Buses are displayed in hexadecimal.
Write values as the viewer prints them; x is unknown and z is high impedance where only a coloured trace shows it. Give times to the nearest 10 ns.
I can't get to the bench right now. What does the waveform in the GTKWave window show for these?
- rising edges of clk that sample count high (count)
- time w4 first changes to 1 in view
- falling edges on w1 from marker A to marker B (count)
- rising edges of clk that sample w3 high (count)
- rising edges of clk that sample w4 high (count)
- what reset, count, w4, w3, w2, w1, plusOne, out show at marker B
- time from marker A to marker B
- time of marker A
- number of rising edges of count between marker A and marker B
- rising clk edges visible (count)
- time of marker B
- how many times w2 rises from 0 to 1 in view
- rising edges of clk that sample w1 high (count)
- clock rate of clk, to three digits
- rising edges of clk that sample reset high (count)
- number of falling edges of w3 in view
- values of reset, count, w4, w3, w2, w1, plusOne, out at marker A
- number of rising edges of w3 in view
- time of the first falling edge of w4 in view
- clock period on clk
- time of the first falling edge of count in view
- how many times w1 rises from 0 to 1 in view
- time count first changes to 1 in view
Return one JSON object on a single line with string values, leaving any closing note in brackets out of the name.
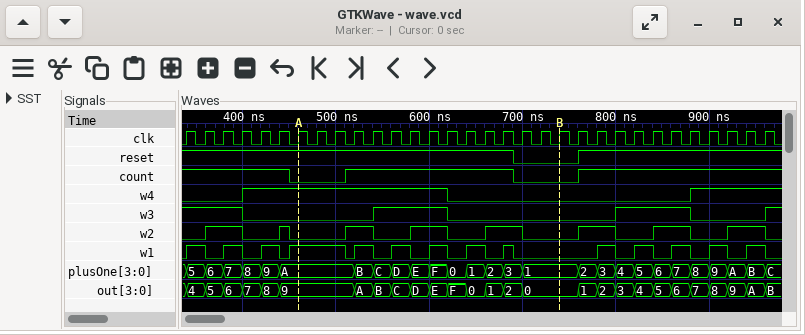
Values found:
{"rising edges of clk that sample count high": "25", "time w4 first changes to 1 in view": "400 ns", "falling edges on w1 from marker A to marker B": "6", "rising edges of clk that sample w3 high": "12", "rising edges of clk that sample w4 high": "15", "what reset, count, w4, w3, w2, w1, plusOne, out show at marker B": "reset=0, count=0, w4=0, w3=0, w2=0, w1=0, plusOne=1, out=0", "time from marker A to marker B": "280 ns", "time of marker A": "460 ns", "number of rising edges of count between marker A and marker B": "1", "rising clk edges visible": "32", "time of marker B": "740 ns", "how many times w2 rises from 0 to 1 in view": "8", "rising edges of clk that sample w1 high": "15", "clock rate of clk, to three digits": "50.0 MHz", "rising edges of clk that sample reset high": "28", "number of falling edges of w3 in view": "3", "values of reset, count, w4, w3, w2, w1, plusOne, out at marker A": "reset=1, count=0, w4=1, w3=0, w2=0, w1=1, plusOne=A, out=9", "number of rising edges of w3 in view": "3", "time of the first falling edge of w4 in view": "620 ns", "clock period on clk": "20 ns", "time of the first falling edge of count in view": "450 ns", "how many times w1 rises from 0 to 1 in view": "14", "time count first changes to 1 in view": "510 ns"}
